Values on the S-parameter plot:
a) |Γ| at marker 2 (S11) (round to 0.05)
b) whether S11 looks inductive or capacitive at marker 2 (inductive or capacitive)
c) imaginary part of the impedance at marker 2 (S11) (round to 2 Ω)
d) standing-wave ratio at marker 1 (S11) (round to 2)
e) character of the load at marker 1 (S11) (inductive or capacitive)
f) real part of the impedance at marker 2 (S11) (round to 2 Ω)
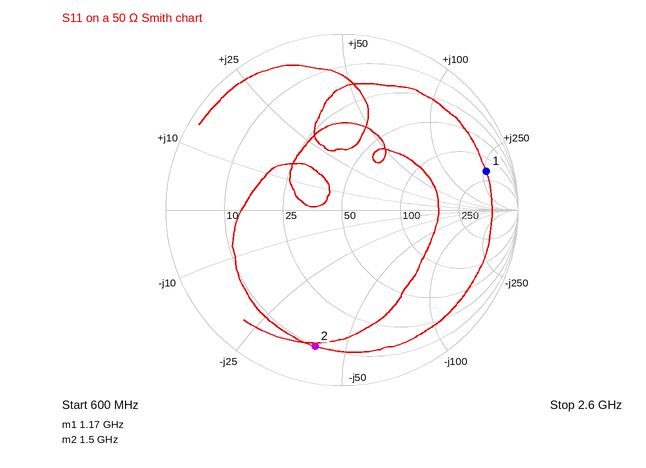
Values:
0.80
capacitive
-40 Ω
12
inductive
10 Ω
